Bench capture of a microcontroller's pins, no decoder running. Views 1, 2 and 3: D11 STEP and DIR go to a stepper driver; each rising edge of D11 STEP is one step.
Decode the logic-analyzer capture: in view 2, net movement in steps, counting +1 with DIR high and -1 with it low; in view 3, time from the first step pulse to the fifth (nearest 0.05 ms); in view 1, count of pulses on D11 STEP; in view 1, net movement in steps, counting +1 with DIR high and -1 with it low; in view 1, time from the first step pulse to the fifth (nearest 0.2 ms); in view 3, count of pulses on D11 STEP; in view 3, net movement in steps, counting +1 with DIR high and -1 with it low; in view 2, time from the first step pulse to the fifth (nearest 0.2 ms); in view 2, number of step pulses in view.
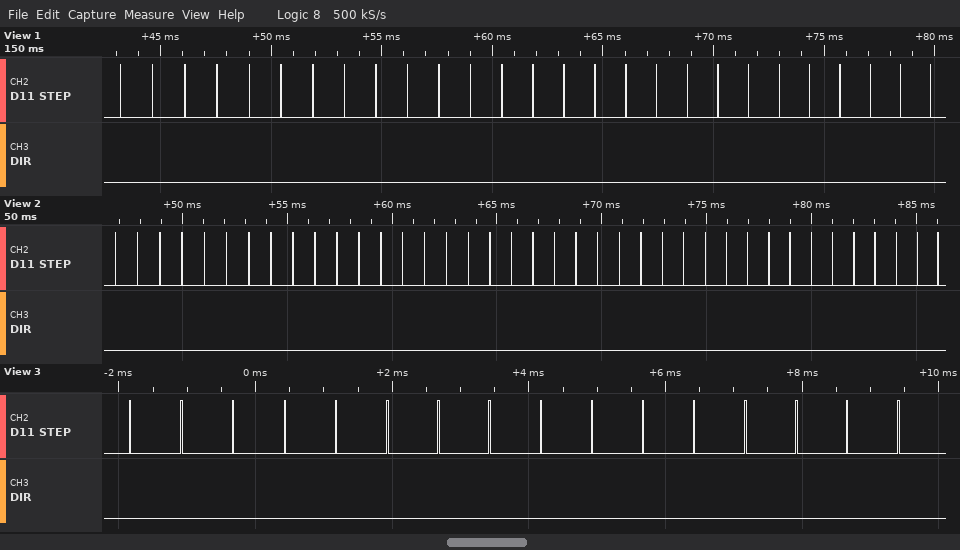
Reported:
-39
3.00 ms
27
-27
5.8 ms
16
-16
4.2 ms
39
